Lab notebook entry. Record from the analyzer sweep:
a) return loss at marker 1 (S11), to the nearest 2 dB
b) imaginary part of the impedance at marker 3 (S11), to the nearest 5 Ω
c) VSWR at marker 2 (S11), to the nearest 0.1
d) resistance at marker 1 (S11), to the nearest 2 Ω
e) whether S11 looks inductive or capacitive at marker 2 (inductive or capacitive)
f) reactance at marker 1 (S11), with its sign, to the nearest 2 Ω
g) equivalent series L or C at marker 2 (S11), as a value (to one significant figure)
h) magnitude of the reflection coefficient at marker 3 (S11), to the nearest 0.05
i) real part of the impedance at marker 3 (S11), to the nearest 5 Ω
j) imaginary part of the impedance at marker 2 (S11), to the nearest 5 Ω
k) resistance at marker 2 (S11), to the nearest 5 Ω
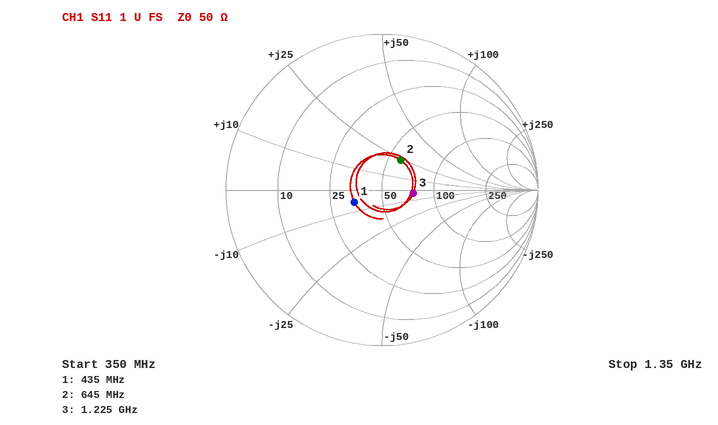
14 dB
-5 Ω
1.6
34 Ω
inductive
-6 Ω
6 nH
0.20
75 Ω
+25 Ω
60 Ω
